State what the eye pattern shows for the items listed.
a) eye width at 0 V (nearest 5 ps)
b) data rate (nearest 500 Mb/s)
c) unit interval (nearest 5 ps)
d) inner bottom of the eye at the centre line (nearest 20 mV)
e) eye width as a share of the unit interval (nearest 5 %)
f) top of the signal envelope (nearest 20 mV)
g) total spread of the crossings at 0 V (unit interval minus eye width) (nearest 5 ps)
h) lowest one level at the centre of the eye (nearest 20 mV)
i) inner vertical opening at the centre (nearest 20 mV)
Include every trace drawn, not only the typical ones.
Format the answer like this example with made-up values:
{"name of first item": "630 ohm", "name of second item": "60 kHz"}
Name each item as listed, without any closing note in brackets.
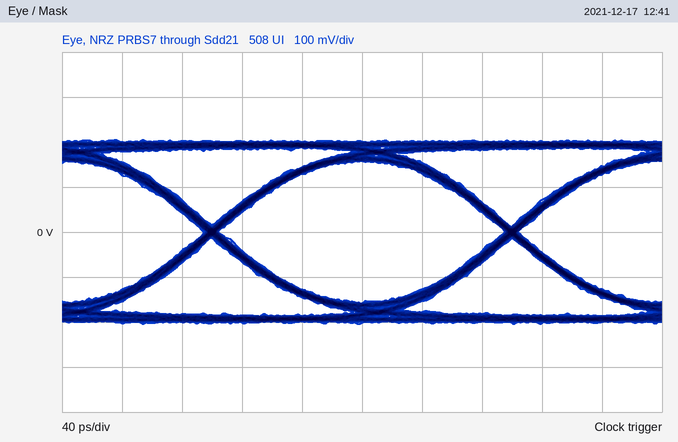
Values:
{"eye width at 0 V": "190 ps", "data rate": "5.0 Gb/s", "unit interval": "200 ps", "inner bottom of the eye at the centre line": "-160 mV", "eye width as a share of the unit interval": "95 %", "top of the signal envelope": "200 mV", "total spread of the crossings at 0 V (unit interval minus eye width)": "10 ps", "lowest one level at the centre of the eye": "160 mV", "inner vertical opening at the centre": "320 mV"}
